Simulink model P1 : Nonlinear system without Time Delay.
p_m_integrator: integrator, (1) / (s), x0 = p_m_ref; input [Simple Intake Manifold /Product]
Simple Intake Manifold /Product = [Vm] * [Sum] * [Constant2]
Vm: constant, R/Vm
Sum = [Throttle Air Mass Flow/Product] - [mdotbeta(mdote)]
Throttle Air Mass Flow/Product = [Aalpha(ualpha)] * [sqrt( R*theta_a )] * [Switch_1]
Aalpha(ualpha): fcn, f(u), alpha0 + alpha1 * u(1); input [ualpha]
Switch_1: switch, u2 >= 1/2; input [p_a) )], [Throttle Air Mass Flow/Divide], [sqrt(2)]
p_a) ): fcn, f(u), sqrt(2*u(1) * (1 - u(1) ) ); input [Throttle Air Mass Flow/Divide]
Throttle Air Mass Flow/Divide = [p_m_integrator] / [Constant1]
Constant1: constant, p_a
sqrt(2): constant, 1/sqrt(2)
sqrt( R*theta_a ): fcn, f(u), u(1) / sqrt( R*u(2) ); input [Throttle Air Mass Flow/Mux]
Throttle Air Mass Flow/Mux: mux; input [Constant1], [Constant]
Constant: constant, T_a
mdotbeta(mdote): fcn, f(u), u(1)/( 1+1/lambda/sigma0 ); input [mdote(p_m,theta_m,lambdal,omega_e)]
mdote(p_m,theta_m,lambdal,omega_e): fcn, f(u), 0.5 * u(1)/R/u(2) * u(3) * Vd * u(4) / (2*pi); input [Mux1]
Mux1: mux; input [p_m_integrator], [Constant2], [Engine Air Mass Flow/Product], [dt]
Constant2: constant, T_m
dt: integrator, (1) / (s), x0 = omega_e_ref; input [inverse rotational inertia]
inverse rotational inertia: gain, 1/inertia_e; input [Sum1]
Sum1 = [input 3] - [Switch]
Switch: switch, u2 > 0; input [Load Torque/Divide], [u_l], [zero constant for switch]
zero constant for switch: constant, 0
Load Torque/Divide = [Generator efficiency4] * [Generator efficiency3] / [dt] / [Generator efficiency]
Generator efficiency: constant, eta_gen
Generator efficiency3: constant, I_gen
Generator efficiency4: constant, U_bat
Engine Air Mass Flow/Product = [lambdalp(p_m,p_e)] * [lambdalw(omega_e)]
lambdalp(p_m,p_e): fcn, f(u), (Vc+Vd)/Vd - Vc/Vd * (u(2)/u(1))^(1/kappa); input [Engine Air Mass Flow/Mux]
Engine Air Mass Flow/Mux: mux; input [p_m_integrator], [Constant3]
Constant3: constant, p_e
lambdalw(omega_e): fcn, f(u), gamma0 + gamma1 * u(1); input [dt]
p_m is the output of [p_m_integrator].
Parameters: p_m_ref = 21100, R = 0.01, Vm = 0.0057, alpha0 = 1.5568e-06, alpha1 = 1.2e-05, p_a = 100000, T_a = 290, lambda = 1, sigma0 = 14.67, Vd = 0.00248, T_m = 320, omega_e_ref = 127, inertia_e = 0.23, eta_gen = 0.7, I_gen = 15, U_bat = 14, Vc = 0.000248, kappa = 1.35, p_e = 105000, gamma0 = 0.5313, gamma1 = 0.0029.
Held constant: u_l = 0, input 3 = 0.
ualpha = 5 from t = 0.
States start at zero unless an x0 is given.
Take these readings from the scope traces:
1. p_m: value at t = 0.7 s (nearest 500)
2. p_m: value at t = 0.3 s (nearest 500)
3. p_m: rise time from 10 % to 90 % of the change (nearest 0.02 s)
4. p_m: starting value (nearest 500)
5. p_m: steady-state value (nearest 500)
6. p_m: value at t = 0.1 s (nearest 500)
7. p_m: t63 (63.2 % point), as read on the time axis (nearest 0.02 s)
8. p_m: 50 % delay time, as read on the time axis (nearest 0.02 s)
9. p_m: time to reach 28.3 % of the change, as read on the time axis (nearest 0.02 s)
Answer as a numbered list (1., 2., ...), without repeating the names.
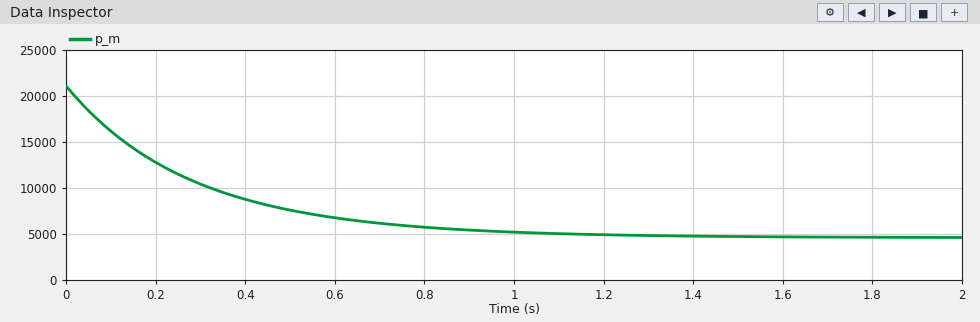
1. 6000
2. 10500
3. 0.66 s
4. 21000
5. 4500
6. 16000
7. 0.28 s
8. 0.20 s
9. 0.10 s
